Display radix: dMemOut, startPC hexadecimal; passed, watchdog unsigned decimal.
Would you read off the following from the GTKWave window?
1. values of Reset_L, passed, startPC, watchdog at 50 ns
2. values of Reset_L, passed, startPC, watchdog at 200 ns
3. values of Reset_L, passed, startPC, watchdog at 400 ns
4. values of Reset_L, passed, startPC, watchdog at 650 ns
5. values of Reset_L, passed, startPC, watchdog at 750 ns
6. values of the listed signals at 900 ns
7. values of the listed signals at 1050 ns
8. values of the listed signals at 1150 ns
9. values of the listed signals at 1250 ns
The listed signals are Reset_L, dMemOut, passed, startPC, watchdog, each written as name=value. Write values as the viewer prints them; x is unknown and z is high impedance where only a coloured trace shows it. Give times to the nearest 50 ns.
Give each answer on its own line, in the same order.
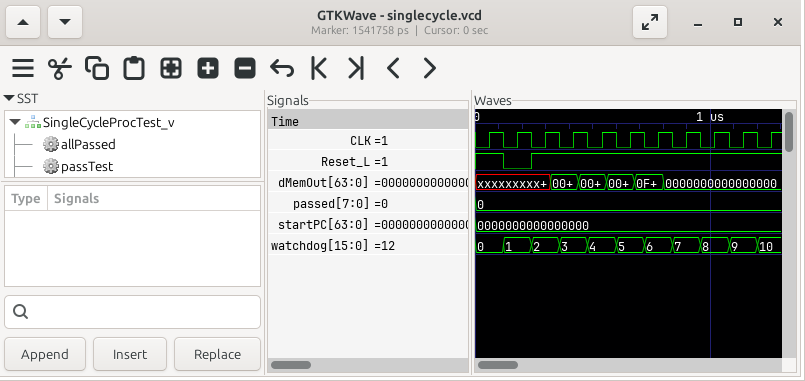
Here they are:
Reset_L=1, passed=0, startPC=0000000000000000, watchdog=0
Reset_L=0, passed=0, startPC=0000000000000000, watchdog=1
Reset_L=1, passed=0, startPC=0000000000000000, watchdog=3
Reset_L=1, passed=0, startPC=0000000000000000, watchdog=5
Reset_L=1, passed=0, startPC=0000000000000000, watchdog=6
Reset_L=1, dMemOut=0000000000000000, passed=0, startPC=0000000000000000, watchdog=7
Reset_L=1, dMemOut=0000000000000000, passed=0, startPC=0000000000000000, watchdog=8
Reset_L=1, dMemOut=0000000000000000, passed=0, startPC=0000000000000000, watchdog=9
Reset_L=1, dMemOut=0000000000000000, passed=0, startPC=0000000000000000, watchdog=10
